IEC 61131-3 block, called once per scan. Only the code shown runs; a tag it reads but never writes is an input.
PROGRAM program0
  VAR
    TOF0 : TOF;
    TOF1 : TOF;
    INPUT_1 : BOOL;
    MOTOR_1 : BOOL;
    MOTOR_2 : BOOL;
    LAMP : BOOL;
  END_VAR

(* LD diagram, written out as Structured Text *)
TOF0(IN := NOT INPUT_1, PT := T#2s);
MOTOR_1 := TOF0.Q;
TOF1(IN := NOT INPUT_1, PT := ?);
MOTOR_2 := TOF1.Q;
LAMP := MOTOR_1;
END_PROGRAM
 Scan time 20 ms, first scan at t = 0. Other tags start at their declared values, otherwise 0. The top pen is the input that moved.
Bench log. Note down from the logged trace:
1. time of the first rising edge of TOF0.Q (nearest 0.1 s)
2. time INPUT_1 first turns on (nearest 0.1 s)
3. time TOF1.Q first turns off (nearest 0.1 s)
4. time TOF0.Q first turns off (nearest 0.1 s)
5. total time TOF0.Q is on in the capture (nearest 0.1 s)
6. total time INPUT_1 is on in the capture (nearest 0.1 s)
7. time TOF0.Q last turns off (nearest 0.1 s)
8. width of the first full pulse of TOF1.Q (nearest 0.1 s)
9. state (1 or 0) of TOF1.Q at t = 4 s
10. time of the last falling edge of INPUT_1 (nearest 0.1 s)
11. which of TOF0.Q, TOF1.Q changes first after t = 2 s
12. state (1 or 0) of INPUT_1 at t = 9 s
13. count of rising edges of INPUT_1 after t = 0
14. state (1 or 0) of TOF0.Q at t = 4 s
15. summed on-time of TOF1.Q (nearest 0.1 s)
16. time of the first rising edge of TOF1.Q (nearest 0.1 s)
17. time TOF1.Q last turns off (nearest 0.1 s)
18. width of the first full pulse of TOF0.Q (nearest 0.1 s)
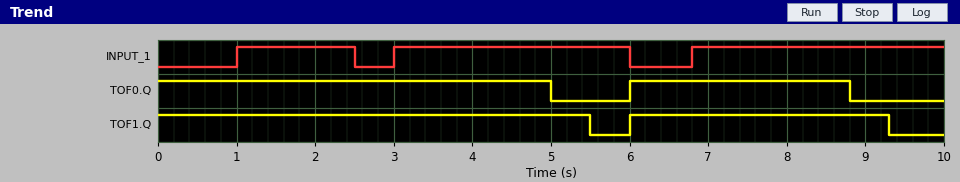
6.0 s
1.0 s
5.5 s
5.0 s
7.8 s
7.7 s
8.8 s
3.3 s
1
6.0 s
TOF0.Q
1
3
1
8.8 s
6.0 s
9.3 s
2.8 s
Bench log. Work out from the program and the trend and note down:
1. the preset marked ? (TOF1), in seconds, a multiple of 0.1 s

2.5 s
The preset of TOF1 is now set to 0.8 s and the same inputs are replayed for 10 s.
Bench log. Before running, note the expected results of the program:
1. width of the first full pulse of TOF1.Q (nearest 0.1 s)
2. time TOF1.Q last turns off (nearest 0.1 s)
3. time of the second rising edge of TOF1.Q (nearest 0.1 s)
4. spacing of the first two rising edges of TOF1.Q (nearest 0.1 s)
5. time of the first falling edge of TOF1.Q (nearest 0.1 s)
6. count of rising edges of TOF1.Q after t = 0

1.3 s
7.6 s
6.0 s
3.5 s
1.8 s
2
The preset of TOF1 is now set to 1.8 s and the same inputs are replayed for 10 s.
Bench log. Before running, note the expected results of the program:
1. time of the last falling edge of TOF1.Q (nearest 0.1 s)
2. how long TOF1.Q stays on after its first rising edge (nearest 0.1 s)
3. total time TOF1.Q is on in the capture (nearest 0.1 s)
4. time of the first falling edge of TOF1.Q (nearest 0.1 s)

8.6 s
2.6 s
7.4 s
4.8 s
